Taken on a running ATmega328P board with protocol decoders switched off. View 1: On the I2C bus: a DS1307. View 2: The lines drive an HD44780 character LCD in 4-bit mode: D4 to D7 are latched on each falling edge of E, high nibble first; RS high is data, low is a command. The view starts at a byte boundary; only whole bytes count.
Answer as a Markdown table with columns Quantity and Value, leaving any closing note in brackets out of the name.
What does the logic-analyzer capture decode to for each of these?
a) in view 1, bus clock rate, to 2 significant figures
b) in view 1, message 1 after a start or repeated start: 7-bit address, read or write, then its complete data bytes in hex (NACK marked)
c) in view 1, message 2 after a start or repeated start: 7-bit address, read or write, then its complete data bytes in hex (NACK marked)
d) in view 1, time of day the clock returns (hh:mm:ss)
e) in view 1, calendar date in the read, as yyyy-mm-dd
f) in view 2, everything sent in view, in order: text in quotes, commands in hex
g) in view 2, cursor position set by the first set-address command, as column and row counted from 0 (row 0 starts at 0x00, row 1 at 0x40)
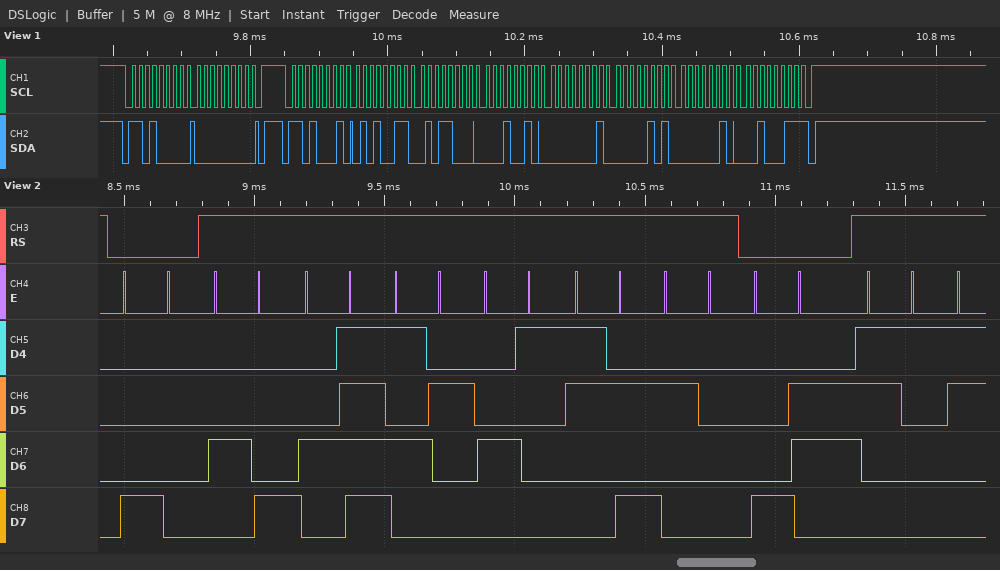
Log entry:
| Quantity | Value |
|---|---|
| in view 1, bus clock rate, to 2 significant figures | 100 kHz |
| in view 1, message 1 after a start or repeated start: 7-bit address, read or write, then its complete data bytes in hex | 0x68 write: 00 |
| in view 1, message 2 after a start or repeated start: 7-bit address, read or write, then its complete data bytes in hex | 0x68 read: 53 58 12 01 05 02 23 NACK |
| in view 1, time of day the clock returns | 12:58:53 |
| in view 1, calendar date in the read, as yyyy-mm-dd | 2023-02-05 |
| in view 2, everything sent in view, in order: text in quotes, commands in hex | 0x80 "HORA: " 0x86 "1" |
| in view 2, cursor position set by the first set-address command, as column and row counted from 0 | column 0, row 0 |
